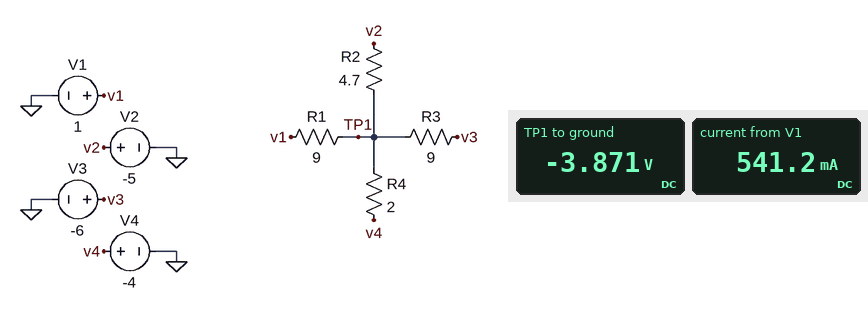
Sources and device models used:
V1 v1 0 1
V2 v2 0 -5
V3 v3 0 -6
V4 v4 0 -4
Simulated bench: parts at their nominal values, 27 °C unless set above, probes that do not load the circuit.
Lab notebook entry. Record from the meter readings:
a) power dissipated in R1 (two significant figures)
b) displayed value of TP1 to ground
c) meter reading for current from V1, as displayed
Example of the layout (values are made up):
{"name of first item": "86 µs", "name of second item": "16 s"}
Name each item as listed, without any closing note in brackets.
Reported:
{"power dissipated in R1": "2.6 W", "displayed value of TP1 to ground": "-3.871 V", "meter reading for current from V1, as displayed": "541.2 mA"}
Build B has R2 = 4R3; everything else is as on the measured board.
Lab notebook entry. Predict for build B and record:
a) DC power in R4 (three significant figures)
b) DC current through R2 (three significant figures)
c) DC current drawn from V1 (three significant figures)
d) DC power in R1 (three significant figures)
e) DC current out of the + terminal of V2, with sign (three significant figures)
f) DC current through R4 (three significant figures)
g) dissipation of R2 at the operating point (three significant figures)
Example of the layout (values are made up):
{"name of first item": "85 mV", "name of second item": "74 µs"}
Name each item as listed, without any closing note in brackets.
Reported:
{"DC power in R4": "5.57 mW", "DC current through R2": "257 mA", "DC current drawn from V1": "544 mA", "DC power in R1": "2.66 W", "DC current out of the + terminal of V2, with sign": "-257 mA", "DC current through R4": "52.8 mA", "dissipation of R2 at the operating point": "284 mW"}
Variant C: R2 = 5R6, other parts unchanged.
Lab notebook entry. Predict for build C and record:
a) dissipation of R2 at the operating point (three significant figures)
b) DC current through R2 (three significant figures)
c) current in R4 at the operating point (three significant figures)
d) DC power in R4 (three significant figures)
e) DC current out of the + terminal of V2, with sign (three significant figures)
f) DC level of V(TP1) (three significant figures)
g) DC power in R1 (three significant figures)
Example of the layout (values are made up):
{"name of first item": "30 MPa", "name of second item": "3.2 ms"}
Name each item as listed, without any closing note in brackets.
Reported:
{"dissipation of R2 at the operating point": "245 mW", "DC current through R2": "209 mA", "current in R4 at the operating point": "85.9 mA", "DC power in R4": "14.8 mW", "DC current out of the + terminal of V2, with sign": "-209 mA", "DC level of V(TP1)": "-3.83 V", "DC power in R1": "2.59 W"}
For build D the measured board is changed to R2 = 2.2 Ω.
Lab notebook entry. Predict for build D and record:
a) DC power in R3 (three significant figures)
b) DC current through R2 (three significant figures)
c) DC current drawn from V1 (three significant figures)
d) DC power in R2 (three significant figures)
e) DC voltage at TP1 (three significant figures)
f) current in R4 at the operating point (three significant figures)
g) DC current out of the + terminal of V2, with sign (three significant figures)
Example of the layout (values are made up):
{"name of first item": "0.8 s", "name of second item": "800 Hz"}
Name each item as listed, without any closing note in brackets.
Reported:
{"DC power in R3": "400 mW", "DC current through R2": "408 mA", "DC current drawn from V1": "567 mA", "DC power in R2": "366 mW", "DC voltage at TP1": "-4.10 V", "current in R4 at the operating point": "51.5 mA", "DC current out of the + terminal of V2, with sign": "-408 mA"}
